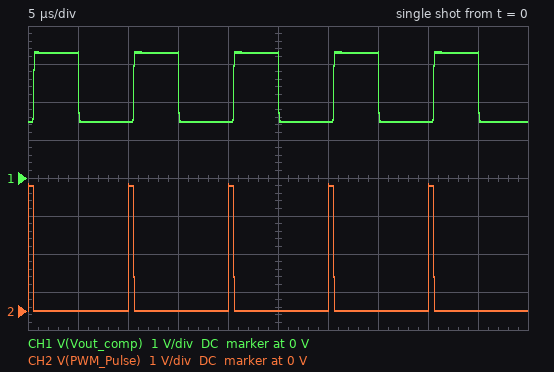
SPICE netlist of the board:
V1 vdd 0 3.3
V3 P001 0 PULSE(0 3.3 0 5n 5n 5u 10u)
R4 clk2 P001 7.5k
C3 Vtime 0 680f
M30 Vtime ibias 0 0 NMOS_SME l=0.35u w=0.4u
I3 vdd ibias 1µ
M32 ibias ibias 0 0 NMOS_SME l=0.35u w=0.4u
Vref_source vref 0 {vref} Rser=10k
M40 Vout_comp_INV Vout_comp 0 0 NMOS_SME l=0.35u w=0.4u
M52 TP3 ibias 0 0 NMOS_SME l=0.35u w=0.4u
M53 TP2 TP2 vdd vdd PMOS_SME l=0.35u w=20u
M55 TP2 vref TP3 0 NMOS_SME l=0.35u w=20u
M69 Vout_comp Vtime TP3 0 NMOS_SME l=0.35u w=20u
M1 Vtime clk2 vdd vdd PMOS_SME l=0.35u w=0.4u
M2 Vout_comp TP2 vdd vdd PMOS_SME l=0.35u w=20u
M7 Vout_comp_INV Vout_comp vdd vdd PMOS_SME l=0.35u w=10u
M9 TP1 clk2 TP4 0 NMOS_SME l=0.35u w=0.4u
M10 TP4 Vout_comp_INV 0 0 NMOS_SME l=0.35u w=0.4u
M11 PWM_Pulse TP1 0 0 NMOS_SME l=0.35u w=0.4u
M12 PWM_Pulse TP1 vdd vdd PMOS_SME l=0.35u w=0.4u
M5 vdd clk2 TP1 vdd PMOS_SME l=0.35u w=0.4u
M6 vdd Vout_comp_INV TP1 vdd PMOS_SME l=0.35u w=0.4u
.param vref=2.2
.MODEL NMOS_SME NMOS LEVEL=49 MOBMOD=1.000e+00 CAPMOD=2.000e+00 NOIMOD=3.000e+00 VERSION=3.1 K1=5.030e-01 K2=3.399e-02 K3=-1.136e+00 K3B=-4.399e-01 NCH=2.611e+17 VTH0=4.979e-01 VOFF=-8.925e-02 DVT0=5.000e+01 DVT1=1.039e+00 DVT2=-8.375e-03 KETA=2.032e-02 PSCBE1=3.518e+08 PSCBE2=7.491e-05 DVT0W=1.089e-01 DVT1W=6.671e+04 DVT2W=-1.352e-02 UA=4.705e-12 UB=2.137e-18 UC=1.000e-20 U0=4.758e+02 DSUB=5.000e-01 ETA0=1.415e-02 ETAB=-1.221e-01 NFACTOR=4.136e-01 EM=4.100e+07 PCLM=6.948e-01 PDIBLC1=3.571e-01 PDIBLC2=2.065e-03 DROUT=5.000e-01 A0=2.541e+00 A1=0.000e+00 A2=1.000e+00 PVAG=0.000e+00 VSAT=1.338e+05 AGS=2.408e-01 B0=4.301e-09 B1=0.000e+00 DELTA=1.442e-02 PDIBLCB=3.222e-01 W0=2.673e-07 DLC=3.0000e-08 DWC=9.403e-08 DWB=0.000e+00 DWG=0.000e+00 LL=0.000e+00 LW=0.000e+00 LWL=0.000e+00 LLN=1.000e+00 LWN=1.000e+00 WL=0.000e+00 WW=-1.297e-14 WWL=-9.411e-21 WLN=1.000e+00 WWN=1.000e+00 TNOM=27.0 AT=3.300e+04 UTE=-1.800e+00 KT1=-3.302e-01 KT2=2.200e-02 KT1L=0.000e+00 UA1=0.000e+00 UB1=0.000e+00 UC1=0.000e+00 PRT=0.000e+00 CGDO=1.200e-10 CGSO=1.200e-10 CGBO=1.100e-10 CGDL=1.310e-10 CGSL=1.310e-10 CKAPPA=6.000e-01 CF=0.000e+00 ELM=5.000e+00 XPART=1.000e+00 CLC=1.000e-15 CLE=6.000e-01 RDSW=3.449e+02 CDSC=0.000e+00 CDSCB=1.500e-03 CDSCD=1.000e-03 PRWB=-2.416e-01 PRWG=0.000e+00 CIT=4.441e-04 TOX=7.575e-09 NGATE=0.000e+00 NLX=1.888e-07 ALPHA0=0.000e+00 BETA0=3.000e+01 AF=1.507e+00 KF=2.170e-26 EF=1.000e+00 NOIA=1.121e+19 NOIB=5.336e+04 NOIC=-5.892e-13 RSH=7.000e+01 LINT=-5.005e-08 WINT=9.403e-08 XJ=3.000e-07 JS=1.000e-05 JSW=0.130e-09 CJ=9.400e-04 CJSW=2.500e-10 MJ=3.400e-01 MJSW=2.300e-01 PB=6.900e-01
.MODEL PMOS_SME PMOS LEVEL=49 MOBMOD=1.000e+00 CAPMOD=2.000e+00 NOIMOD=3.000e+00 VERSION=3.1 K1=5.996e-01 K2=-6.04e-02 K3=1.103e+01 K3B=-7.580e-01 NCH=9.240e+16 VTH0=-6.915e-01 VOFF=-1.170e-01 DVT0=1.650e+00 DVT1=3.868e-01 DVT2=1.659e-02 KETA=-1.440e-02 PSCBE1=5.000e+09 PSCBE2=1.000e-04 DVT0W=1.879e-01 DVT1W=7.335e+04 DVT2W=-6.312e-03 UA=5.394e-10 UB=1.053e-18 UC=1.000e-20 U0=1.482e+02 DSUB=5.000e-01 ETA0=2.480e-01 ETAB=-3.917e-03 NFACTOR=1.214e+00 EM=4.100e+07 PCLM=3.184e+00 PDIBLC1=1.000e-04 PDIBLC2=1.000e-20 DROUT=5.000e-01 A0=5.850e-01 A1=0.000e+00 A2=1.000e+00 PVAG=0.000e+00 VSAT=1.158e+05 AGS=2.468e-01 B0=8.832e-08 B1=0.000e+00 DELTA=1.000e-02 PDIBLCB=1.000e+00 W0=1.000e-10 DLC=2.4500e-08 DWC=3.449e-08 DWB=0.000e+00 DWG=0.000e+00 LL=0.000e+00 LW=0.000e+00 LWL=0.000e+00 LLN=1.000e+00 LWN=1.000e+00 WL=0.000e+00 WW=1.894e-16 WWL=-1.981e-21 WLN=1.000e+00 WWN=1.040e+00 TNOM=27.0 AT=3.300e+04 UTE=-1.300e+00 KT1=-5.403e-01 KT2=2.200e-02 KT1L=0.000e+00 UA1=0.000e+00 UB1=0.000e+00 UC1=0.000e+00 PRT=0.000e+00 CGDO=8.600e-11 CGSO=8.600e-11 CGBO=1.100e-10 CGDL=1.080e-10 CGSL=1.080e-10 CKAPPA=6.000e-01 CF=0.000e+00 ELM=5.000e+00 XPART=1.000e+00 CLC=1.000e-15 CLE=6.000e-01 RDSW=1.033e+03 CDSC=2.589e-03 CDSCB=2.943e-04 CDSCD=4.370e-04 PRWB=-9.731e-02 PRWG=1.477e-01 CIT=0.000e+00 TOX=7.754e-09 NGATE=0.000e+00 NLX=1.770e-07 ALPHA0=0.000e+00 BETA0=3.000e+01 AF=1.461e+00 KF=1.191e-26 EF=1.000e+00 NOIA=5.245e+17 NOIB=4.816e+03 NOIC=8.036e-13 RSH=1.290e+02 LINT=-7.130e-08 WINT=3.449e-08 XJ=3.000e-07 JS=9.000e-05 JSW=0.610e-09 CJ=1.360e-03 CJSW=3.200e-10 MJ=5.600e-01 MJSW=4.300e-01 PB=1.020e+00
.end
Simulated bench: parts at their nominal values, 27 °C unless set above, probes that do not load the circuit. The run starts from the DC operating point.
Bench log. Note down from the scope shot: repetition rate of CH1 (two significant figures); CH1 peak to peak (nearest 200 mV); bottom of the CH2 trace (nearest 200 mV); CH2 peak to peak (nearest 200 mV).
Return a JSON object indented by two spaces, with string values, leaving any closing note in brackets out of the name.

{
  "repetition rate of CH1": "100 kHz",
  "CH1 peak to peak": "1.8 V",
  "bottom of the CH2 trace": "0 V",
  "CH2 peak to peak": "3.4 V"
}
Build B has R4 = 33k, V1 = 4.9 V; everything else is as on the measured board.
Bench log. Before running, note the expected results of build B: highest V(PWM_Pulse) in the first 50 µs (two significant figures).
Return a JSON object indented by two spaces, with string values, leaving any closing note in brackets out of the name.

{
  "highest V(PWM_Pulse) in the first 50 µs": "4.9 V"
}
